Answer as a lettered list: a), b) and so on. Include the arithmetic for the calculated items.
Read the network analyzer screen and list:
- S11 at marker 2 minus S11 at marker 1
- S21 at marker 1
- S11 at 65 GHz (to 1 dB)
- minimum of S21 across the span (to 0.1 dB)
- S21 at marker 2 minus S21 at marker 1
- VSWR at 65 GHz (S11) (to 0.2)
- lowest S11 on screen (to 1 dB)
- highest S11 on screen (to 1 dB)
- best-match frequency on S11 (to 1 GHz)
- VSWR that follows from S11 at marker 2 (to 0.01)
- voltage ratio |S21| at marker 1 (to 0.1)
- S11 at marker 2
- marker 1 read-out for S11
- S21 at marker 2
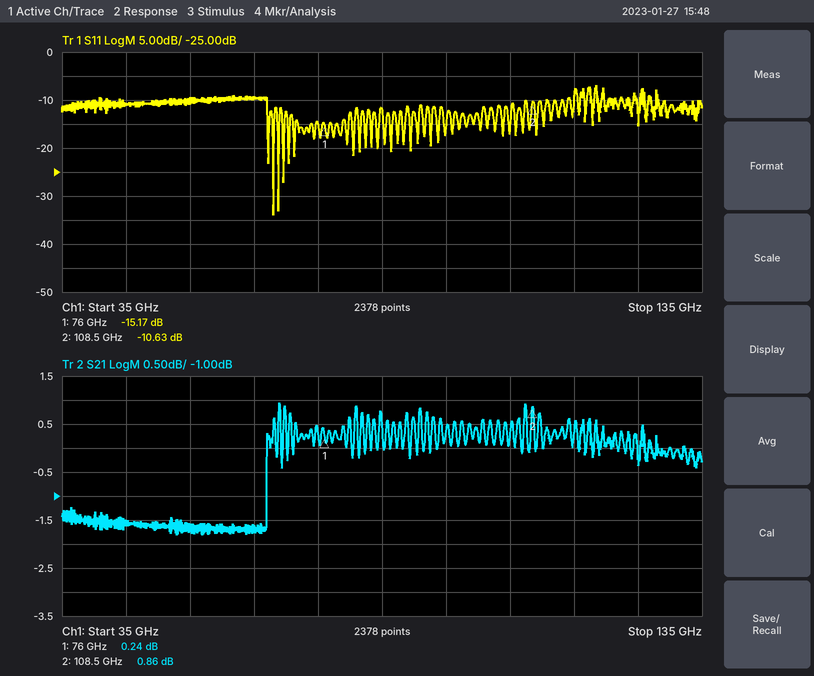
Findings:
a) -10.63 − (-15.17) = 4.54 dB
b) 0.24 dB
c) -10 dB
d) -1.8 dB
e) 0.86 − (0.24) = 0.62 dB
f) |Γ| = 10^(-10/20) = 0.3162; VSWR = (1 + 0.3162)/(1 − 0.3162) ≈ 1.92, so 2.0 to the nearest 0.2
g) -34 dB
h) -7 dB
i) 68 GHz
j) (1 + 0.2941)/(1 − 0.2941) ≈ 1.83
k) 10^(0.24/20) ≈ 1.0
l) -10.63 dB
m) -15.17 dB
n) 0.86 dB
